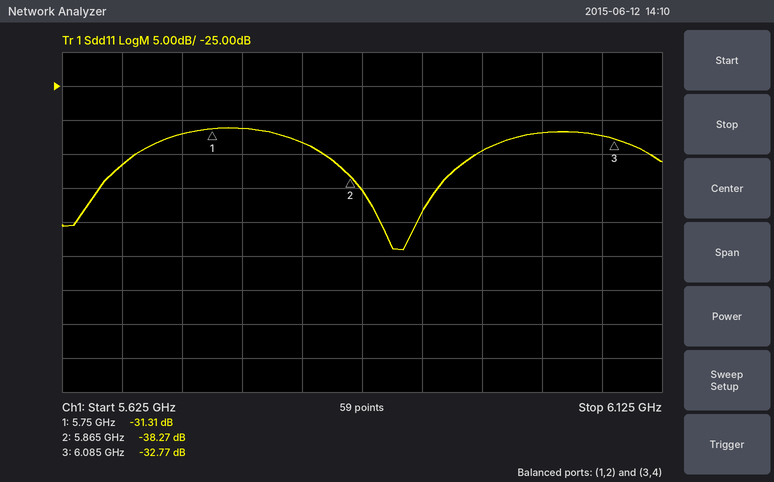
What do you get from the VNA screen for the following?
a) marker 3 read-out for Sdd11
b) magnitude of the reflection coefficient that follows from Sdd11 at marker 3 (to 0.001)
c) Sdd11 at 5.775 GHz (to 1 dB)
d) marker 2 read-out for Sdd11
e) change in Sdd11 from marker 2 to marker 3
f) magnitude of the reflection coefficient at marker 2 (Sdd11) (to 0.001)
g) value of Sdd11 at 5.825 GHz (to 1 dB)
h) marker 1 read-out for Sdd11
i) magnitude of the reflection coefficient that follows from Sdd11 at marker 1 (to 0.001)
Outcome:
-32.77 dB
0.023
-31 dB
-38.27 dB
5.50 dB
0.012
-33 dB
-31.31 dB
0.027
